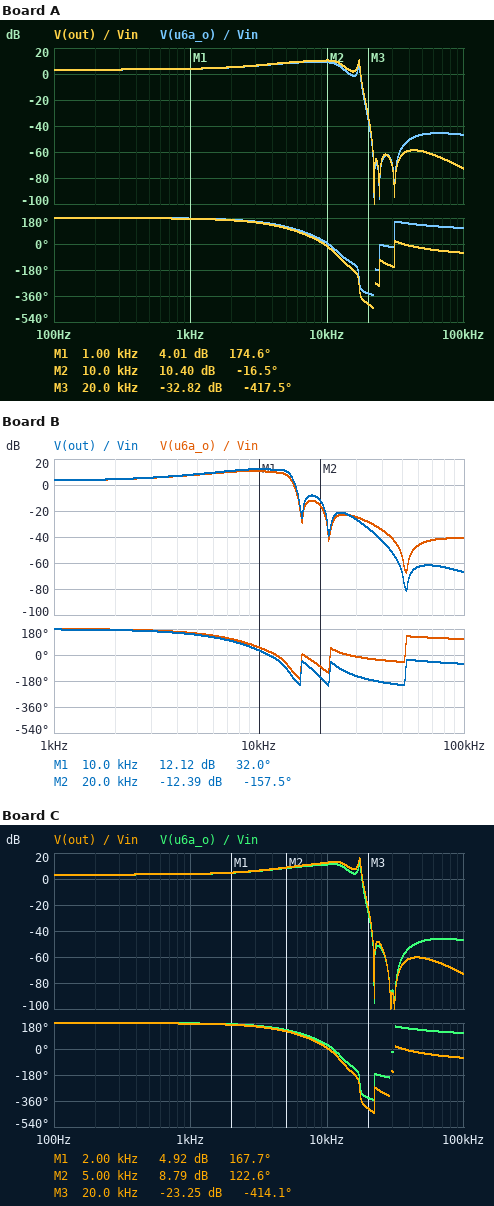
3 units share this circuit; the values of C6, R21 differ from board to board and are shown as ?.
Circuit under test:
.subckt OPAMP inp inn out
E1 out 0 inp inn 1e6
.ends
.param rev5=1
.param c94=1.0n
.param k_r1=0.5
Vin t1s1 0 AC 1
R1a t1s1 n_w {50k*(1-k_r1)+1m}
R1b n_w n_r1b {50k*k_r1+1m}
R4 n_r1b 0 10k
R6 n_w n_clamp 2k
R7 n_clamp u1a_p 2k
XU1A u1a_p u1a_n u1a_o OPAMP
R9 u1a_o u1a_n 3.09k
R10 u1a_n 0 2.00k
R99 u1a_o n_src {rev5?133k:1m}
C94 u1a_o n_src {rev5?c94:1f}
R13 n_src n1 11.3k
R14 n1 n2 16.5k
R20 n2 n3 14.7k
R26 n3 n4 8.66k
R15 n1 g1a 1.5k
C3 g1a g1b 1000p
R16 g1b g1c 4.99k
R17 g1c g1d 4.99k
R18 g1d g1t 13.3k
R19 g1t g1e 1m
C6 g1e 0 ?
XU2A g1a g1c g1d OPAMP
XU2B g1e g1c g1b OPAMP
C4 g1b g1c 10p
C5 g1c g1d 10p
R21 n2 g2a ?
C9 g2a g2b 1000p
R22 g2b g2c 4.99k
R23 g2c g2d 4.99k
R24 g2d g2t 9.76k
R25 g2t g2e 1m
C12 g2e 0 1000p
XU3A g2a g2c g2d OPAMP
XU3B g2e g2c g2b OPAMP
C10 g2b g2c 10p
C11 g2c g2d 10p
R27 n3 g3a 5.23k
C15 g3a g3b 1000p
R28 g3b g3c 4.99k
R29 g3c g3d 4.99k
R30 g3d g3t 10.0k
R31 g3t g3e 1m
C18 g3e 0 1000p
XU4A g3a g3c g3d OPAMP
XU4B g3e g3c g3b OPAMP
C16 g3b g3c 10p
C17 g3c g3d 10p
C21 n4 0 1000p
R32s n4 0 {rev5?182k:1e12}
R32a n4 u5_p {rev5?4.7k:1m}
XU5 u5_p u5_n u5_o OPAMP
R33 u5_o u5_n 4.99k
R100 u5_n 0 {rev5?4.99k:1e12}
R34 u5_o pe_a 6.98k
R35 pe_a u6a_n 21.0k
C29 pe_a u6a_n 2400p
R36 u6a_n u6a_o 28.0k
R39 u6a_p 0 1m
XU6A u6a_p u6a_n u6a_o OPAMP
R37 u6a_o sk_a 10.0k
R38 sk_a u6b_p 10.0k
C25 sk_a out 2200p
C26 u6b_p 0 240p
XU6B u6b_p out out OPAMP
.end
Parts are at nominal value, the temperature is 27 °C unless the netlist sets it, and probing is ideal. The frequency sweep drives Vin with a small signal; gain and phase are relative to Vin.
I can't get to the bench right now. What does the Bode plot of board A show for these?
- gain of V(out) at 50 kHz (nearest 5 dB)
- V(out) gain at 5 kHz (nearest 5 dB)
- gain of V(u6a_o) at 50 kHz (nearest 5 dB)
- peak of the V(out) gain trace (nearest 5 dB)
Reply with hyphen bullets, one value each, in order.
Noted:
- -60 dB
- 10 dB
- -45 dB
- 10 dB
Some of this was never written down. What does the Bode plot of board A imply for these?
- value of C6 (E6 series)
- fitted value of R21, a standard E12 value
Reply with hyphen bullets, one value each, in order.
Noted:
- 2.2 nF
- 2.7 kΩ
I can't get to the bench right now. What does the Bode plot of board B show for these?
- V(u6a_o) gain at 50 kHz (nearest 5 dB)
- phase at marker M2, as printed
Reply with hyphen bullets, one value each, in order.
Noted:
- -55 dB
- -157.5 deg
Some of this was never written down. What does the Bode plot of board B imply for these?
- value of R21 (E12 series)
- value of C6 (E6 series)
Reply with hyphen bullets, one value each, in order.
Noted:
- 10 kΩ
- 470 pF
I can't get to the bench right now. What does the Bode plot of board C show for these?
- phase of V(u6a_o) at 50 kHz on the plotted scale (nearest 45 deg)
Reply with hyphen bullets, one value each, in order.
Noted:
- 135 deg
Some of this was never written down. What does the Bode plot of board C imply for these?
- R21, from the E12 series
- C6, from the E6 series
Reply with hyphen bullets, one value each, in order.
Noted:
- 2.7 kΩ
- 1.5 nF
